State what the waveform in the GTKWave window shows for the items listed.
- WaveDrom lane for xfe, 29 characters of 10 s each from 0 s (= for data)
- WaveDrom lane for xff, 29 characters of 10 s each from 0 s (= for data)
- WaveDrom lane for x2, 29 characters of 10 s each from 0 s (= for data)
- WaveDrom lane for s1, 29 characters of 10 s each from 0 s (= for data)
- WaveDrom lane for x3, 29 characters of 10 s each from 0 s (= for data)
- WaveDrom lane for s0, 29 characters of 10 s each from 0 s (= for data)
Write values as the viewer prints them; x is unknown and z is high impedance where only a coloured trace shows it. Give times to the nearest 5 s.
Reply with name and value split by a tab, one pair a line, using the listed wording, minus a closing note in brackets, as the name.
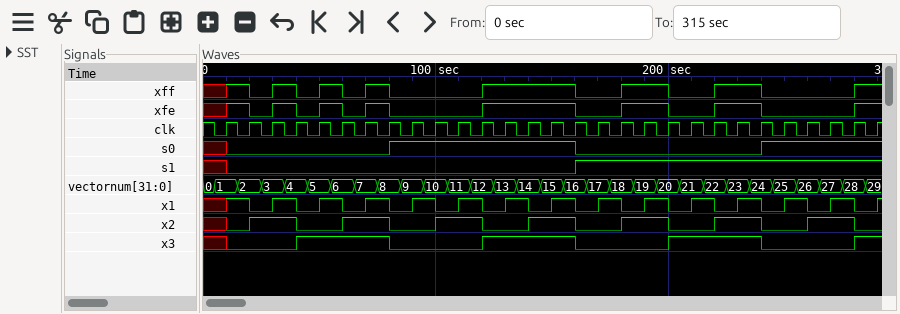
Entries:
WaveDrom lane for xfe, 29 characters of 10 s each from 0 s	{name: 'xfe', wave: 'x10101010...1...0.1.0.1.0...1'}
WaveDrom lane for xff, 29 characters of 10 s each from 0 s	{name: 'xff', wave: 'x10101010...1...0.1.0.1.0...1'}
WaveDrom lane for x2, 29 characters of 10 s each from 0 s	{name: 'x2', wave: 'x01.0.1.0.1.0.1.0.1.0.1.0.1.0'}
WaveDrom lane for s1, 29 characters of 10 s each from 0 s	{name: 's1', wave: 'x0..............1............'}
WaveDrom lane for x3, 29 characters of 10 s each from 0 s	{name: 'x3', wave: 'x0..1...0...1...0...1...0...1'}
WaveDrom lane for s0, 29 characters of 10 s each from 0 s	{name: 's0', wave: 'x0......1.......0.......1....'}
